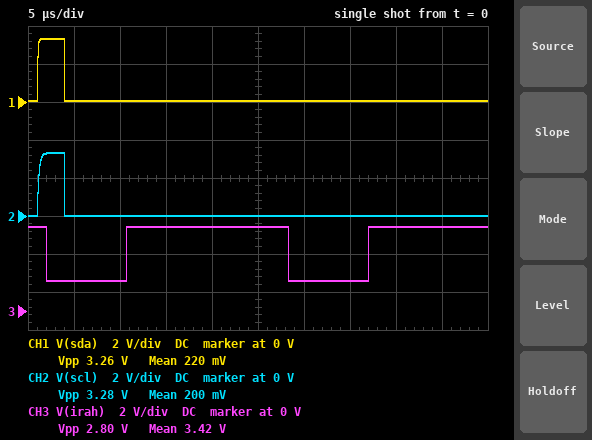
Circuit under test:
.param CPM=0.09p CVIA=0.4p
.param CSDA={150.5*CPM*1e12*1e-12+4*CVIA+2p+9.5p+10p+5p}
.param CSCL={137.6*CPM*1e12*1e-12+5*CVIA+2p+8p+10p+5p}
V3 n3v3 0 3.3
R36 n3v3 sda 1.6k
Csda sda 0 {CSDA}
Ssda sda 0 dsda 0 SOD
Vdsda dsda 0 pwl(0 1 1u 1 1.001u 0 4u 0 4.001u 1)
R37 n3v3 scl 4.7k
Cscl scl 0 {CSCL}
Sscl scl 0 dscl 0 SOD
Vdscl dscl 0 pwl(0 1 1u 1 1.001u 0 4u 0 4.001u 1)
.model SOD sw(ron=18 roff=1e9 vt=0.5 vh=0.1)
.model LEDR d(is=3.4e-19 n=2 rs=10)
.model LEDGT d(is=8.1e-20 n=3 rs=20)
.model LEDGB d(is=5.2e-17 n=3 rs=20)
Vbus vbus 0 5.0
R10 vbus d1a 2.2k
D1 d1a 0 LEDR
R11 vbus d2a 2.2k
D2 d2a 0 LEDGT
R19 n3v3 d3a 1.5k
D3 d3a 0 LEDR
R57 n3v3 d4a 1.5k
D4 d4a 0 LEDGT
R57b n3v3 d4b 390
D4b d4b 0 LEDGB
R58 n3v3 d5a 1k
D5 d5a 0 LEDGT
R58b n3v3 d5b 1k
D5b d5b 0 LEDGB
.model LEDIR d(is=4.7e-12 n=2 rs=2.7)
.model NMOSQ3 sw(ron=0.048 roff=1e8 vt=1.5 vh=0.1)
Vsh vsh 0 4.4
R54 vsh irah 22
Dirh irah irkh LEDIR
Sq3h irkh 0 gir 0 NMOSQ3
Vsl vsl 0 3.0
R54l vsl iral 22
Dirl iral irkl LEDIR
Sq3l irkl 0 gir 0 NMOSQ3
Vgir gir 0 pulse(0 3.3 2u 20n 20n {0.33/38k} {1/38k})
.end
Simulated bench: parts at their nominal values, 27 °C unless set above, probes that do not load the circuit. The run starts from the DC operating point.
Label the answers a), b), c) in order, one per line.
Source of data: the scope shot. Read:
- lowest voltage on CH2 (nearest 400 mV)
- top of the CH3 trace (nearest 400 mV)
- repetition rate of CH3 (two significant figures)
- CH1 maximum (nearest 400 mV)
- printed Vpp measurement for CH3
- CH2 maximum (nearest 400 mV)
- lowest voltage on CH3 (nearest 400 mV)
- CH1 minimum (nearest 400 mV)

a) 0 V
b) 4.4 V
c) 38 kHz
d) 3.2 V
e) 2.80 V
f) 3.2 V
g) 1.6 V
h) 0 V
